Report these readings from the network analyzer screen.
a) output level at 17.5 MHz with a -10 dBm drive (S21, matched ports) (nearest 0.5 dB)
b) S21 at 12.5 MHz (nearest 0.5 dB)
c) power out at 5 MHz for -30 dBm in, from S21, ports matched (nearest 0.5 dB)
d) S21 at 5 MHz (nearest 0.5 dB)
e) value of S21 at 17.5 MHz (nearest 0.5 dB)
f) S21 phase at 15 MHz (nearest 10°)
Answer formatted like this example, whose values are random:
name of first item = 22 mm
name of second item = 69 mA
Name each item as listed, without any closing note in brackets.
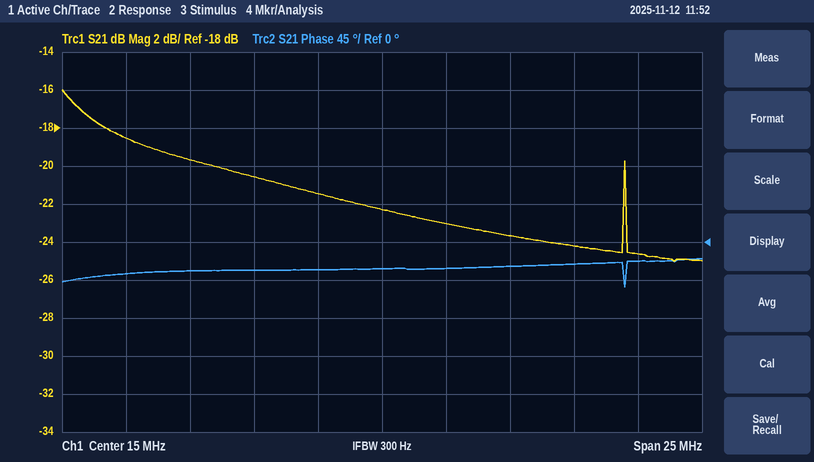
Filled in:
output level at 17.5 MHz with a -10 dBm drive (S21, matched ports) = -33.0 dBm
S21 at 12.5 MHz = -21.5 dB
power out at 5 MHz for -30 dBm in, from S21, ports matched = -48.5 dBm
S21 at 5 MHz = -18.5 dB
value of S21 at 17.5 MHz = -23.0 dB
S21 phase at 15 MHz = -30°
